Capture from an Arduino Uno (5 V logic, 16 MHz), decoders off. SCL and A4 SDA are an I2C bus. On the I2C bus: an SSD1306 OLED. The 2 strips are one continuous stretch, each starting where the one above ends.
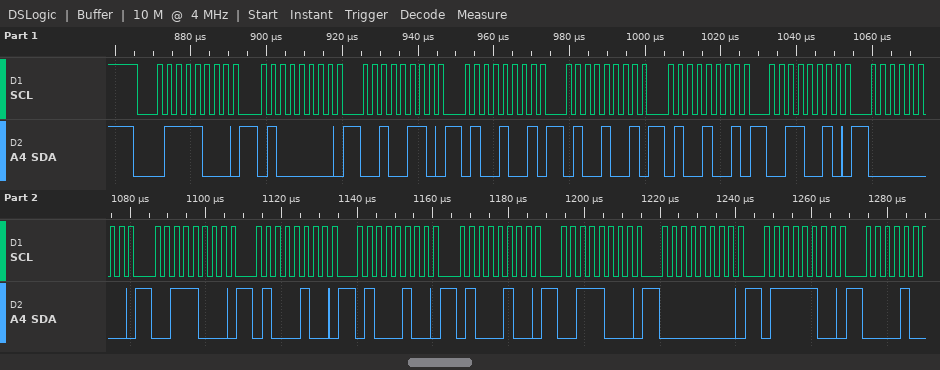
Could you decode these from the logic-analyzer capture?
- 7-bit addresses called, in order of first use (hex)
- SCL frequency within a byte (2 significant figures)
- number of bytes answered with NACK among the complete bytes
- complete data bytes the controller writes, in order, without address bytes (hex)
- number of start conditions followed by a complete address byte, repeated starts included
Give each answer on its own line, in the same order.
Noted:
0x3C
400 kHz
0
40 26 49 49 49 32 00 38 44 44 44 38 00 7C
1
